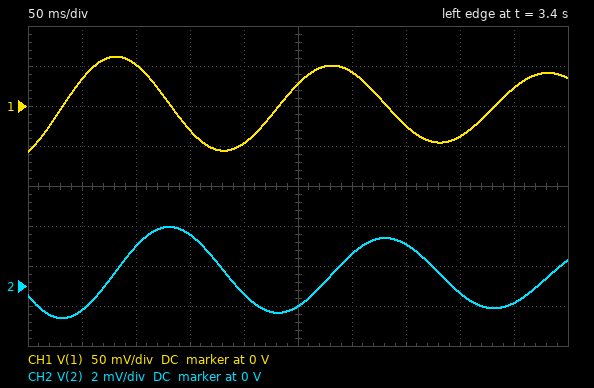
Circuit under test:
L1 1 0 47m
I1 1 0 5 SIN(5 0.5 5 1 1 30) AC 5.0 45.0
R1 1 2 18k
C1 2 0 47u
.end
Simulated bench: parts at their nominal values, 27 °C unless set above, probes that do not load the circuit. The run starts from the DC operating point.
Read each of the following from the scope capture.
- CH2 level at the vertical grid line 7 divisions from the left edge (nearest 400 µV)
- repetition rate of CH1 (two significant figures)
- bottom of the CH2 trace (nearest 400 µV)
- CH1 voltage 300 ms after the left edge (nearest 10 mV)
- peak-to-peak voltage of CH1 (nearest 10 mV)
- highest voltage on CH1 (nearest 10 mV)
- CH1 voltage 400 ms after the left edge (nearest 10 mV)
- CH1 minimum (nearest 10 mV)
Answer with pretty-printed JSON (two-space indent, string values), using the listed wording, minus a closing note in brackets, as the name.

{
  "CH2 level at the vertical grid line 7 divisions from the left edge": "2.0 mV",
  "repetition rate of CH1": "5.0 Hz",
  "bottom of the CH2 trace": "-1.6 mV",
  "CH1 voltage 300 ms after the left edge": "40 mV",
  "peak-to-peak voltage of CH1": "120 mV",
  "highest voltage on CH1": "60 mV",
  "CH1 voltage 400 ms after the left edge": "-40 mV",
  "CH1 minimum": "-60 mV"
}
